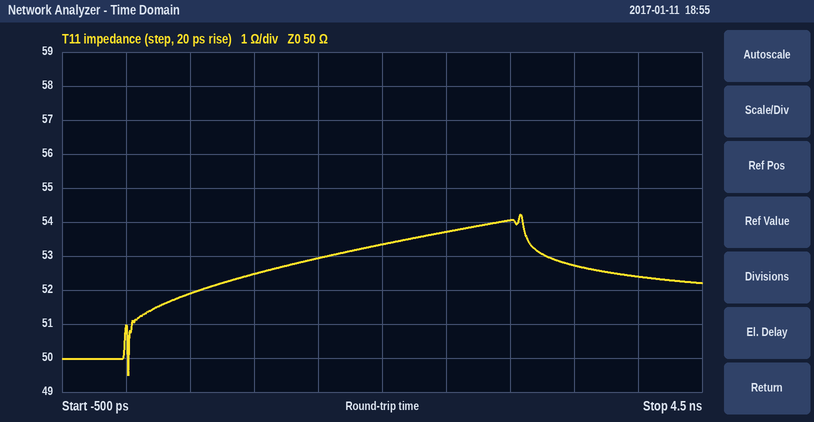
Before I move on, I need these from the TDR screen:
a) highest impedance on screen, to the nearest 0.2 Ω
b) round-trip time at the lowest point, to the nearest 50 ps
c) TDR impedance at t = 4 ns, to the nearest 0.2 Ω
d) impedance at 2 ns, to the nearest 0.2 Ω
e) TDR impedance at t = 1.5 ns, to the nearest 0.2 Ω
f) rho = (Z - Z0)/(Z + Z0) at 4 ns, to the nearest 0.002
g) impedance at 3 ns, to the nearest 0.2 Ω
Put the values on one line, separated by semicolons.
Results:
54.2 Ω; 0 ps; 52.4 Ω; 53.4 Ω; 53.0 Ω; +0.024; 54.0 Ω
